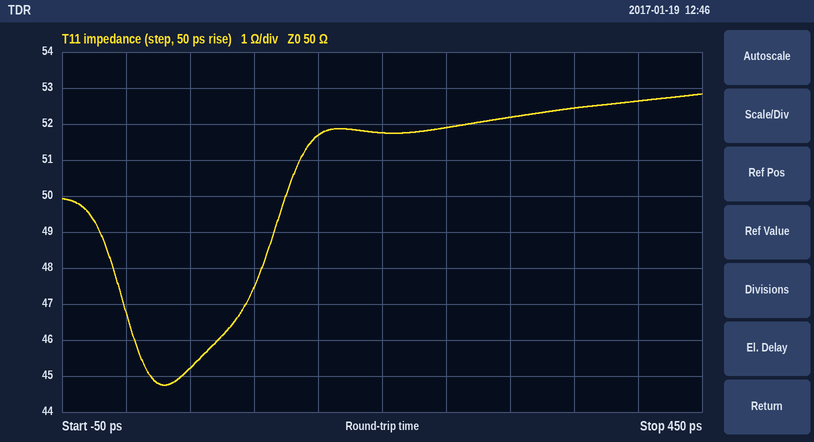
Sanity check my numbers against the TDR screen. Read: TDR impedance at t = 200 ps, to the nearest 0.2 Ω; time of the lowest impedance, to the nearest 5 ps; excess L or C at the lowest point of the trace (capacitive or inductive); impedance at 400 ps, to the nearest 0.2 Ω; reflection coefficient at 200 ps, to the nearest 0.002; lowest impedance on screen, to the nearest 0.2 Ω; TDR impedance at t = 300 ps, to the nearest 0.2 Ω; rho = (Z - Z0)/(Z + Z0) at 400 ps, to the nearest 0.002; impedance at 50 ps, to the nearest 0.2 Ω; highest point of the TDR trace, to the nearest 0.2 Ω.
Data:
51.8 Ω
30 ps
capacitive
52.6 Ω
+0.018
44.8 Ω
52.2 Ω
+0.026
45.2 Ω
52.8 Ω
